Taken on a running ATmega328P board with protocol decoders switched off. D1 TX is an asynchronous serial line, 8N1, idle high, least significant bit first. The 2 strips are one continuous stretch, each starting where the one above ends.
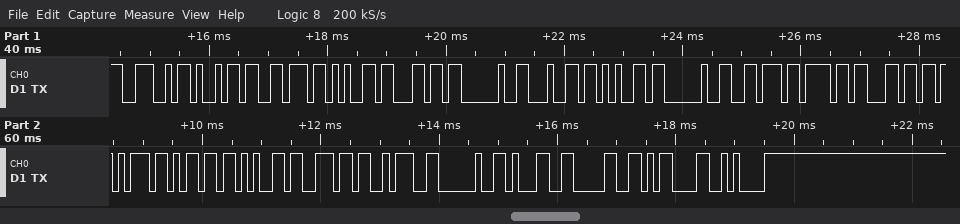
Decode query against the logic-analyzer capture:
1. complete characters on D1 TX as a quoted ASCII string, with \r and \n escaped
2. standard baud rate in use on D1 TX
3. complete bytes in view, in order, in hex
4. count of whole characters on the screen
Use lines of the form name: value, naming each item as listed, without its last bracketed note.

complete characters on D1 TX as a quoted ASCII string, with \r and \n escaped: "Nivel de volumen: 10\r\n"
standard baud rate in use on D1 TX: 9600 baud
complete bytes in view, in order, in hex: 0x4E 0x69 0x76 0x65 0x6C 0x20 0x64 0x65 0x20 0x76 0x6F 0x6C 0x75 0x6D 0x65 0x6E 0x3A 0x20 0x31 0x30 0x0D 0x0A
count of whole characters on the screen: 22
